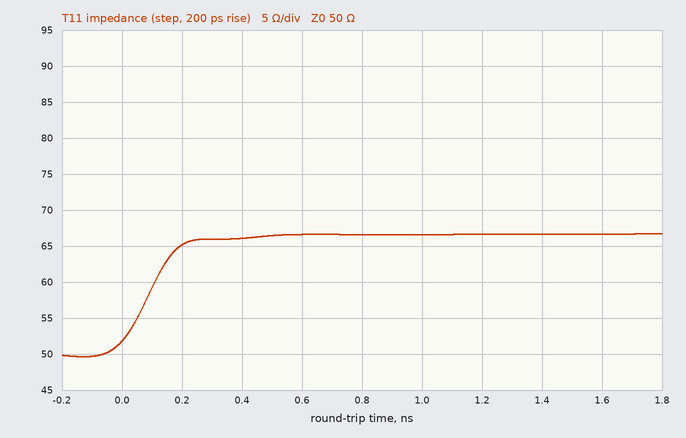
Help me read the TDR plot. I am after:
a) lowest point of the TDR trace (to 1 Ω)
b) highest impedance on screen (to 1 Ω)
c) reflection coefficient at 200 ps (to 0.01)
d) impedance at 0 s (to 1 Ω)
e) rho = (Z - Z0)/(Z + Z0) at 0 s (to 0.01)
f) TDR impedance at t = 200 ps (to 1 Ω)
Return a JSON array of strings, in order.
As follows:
["50 Ω", "67 Ω", "+0.13", "52 Ω", "+0.02", "65 Ω"]
